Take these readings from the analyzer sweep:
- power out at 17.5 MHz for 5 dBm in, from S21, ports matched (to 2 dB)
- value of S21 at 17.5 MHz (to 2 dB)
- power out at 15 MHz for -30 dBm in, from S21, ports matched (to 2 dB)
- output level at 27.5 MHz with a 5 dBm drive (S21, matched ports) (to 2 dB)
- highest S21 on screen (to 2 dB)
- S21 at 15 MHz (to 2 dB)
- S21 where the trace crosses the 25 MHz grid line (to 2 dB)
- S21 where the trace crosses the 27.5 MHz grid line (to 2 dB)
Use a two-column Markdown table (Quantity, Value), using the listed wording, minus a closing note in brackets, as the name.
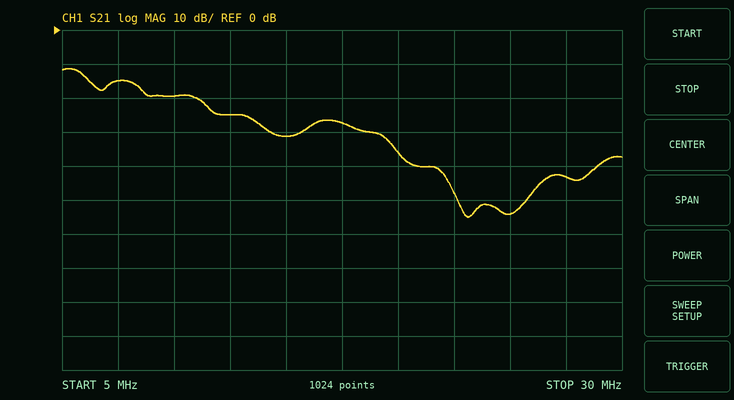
| Quantity | Value |
|---|---|
| power out at 17.5 MHz for 5 dBm in, from S21, ports matched | -22 dBm |
| value of S21 at 17.5 MHz | -28 dB |
| power out at 15 MHz for -30 dBm in, from S21, ports matched | -62 dBm |
| output level at 27.5 MHz with a 5 dBm drive (S21, matched ports) | -38 dBm |
| highest S21 on screen | -12 dB |
| S21 at 15 MHz | -32 dB |
| S21 where the trace crosses the 25 MHz grid line | -54 dB |
| S21 where the trace crosses the 27.5 MHz grid line | -44 dB |
